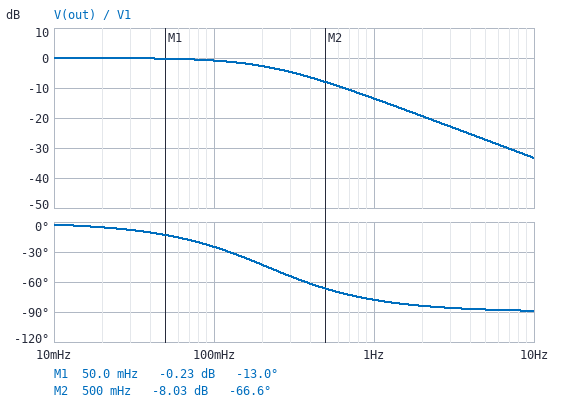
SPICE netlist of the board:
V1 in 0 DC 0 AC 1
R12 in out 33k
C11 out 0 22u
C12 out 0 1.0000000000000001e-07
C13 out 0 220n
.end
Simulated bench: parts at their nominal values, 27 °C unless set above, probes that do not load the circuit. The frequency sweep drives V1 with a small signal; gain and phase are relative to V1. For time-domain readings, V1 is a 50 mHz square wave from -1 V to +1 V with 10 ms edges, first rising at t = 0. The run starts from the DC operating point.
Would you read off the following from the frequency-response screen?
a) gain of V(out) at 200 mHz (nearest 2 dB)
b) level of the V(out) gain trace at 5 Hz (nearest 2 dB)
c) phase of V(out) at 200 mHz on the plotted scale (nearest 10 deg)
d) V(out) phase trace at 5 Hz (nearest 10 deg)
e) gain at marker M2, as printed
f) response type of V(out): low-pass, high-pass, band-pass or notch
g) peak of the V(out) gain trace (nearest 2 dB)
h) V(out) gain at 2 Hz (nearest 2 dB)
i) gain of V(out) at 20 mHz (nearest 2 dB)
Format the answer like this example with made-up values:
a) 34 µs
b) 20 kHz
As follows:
a) -2 dB
b) -28 dB
c) -40 deg
d) -90 deg
e) -8.03 dB
f) low-pass
g) 0 dB
h) -20 dB
i) 0 dB
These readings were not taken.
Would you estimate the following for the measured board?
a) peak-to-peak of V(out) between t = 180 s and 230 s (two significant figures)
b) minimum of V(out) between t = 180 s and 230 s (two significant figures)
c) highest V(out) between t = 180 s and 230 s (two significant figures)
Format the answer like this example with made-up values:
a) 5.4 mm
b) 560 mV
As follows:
a) 2.0 V
b) -1.0 V
c) 1.0 V
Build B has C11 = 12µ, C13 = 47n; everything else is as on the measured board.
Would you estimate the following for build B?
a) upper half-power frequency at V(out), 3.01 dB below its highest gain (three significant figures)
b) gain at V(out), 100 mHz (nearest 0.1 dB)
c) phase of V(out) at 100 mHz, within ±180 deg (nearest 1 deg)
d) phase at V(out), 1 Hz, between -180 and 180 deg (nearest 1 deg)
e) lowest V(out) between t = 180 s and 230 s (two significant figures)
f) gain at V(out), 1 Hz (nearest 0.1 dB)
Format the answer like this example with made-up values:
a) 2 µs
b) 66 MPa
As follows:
a) 397 mHz
b) -0.3 dB
c) -14 deg
d) -68 deg
e) -1.0 V
f) -8.7 dB
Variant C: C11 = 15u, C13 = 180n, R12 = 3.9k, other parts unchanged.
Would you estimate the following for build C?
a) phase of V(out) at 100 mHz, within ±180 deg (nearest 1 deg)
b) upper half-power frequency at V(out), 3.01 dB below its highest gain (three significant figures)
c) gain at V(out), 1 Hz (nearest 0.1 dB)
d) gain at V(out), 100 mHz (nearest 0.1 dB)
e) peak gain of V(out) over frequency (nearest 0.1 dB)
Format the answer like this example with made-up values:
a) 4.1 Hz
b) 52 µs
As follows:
a) -2 deg
b) 2.67 Hz
c) -0.6 dB
d) 0 dB
e) 0 dB
